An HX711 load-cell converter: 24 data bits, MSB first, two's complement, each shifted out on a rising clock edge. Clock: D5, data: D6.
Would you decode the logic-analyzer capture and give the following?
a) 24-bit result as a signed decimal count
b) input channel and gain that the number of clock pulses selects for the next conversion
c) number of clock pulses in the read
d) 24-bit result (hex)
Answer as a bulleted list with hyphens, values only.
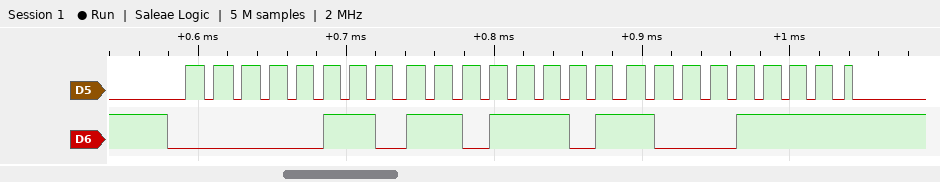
- 449935
- channel A, gain 128
- 25
- 0x06DD8F
